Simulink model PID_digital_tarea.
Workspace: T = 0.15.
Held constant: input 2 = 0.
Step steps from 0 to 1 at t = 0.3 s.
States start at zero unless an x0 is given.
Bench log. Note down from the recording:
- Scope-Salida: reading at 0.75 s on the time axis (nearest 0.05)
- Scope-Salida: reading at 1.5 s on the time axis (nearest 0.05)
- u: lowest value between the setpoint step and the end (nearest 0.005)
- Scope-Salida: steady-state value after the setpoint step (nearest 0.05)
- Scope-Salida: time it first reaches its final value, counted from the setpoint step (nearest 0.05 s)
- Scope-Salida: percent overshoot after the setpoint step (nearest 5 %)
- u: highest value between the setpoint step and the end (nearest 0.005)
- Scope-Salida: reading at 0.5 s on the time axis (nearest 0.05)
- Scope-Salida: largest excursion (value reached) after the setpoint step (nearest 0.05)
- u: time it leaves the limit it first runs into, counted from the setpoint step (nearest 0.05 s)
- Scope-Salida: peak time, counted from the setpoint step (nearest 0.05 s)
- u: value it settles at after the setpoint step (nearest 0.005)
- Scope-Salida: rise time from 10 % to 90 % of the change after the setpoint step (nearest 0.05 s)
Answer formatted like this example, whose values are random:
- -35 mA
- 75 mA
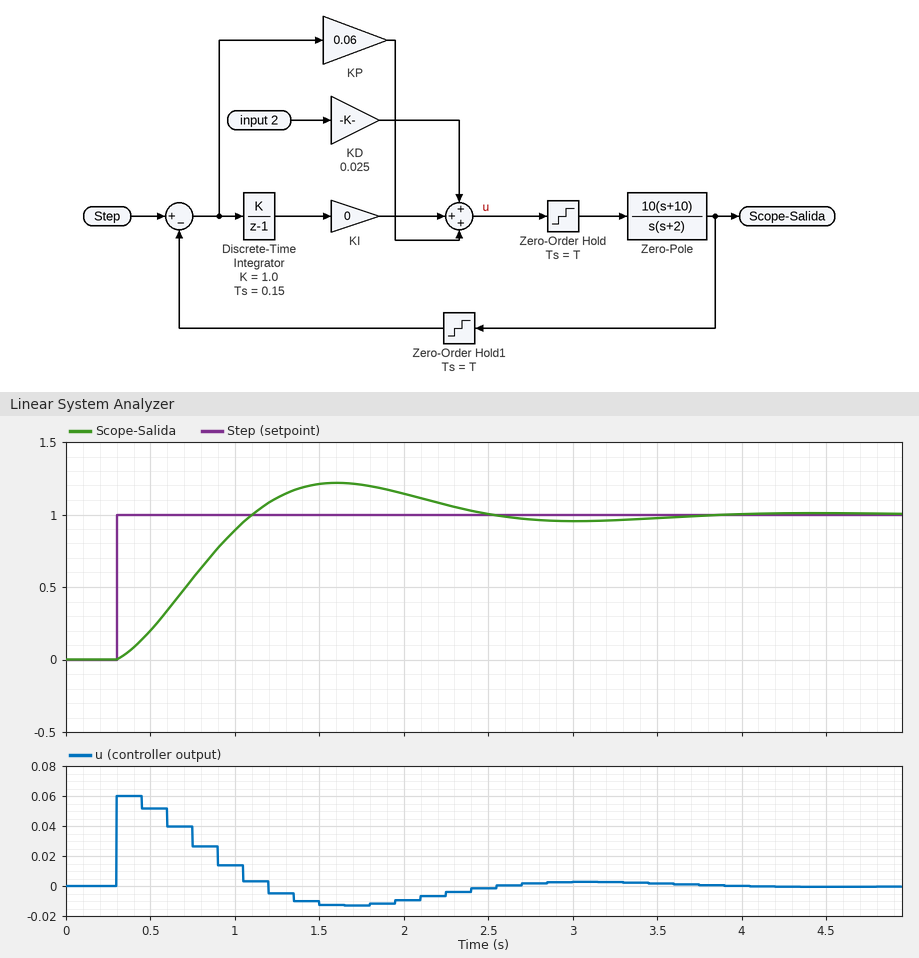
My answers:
- 0.55
- 1.20
- -0.015
- 1.00
- 0.80 s
- 20 %
- 0.060
- 0.20
- 1.20
- 0.15 s
- 1.30 s
- 0.000
- 0.60 s
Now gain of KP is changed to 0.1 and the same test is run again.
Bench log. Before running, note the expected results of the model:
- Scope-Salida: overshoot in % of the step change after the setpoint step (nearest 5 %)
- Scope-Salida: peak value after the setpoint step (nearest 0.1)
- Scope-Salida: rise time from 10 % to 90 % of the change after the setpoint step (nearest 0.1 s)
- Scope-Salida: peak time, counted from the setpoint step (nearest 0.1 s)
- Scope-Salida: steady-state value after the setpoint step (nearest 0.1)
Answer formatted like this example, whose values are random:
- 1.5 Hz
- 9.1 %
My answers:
- 30 %
- 1.3
- 0.4 s
- 0.9 s
- 1.0
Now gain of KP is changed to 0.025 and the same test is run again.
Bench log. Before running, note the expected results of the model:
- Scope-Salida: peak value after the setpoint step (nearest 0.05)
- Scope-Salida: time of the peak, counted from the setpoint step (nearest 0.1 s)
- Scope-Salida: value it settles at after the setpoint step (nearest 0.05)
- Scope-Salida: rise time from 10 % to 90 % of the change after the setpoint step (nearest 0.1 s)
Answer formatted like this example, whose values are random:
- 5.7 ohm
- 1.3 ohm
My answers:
- 1.05
- 2.5 s
- 1.00
- 1.2 s
